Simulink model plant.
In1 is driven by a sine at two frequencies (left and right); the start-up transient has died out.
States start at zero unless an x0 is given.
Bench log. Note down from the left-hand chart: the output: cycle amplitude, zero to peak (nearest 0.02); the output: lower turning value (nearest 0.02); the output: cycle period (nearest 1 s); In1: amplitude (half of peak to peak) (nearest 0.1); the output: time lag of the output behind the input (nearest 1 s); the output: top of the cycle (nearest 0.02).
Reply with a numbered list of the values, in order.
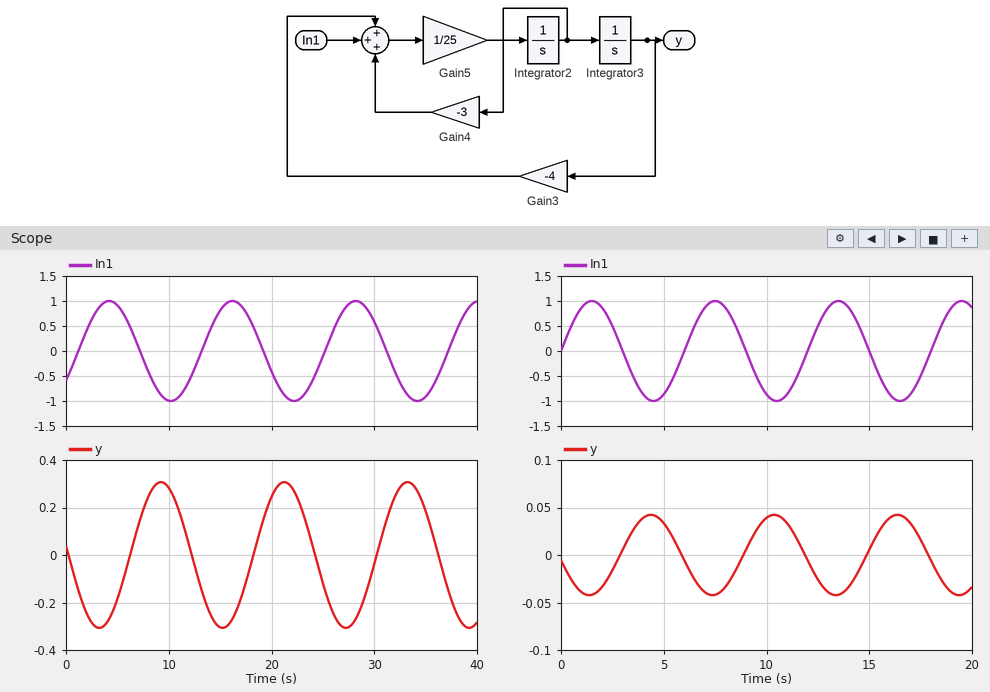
1. 0.30
2. -0.30
3. 12 s
4. 1.0
5. 5 s
6. 0.30
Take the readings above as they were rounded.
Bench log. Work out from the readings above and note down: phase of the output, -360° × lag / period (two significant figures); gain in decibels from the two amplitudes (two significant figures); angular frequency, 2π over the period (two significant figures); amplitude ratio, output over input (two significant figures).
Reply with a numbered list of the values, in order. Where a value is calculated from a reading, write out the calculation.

1. -360 × 5 / 12 = -150°
2. 20 log10(0.3 / 1) = -10 dB
3. 2π / 12 = 0.52 rad/s
4. 0.3 / 1 = 0.30
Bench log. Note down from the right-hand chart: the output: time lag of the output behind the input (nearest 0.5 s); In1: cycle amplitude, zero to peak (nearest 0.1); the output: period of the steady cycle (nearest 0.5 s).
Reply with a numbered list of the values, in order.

1. 3.0 s
2. 1.0
3. 6.0 s
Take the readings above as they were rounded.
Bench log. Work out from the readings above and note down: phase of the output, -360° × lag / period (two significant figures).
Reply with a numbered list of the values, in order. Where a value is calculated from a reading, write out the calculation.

1. -360 × 3 / 6 = -180°
